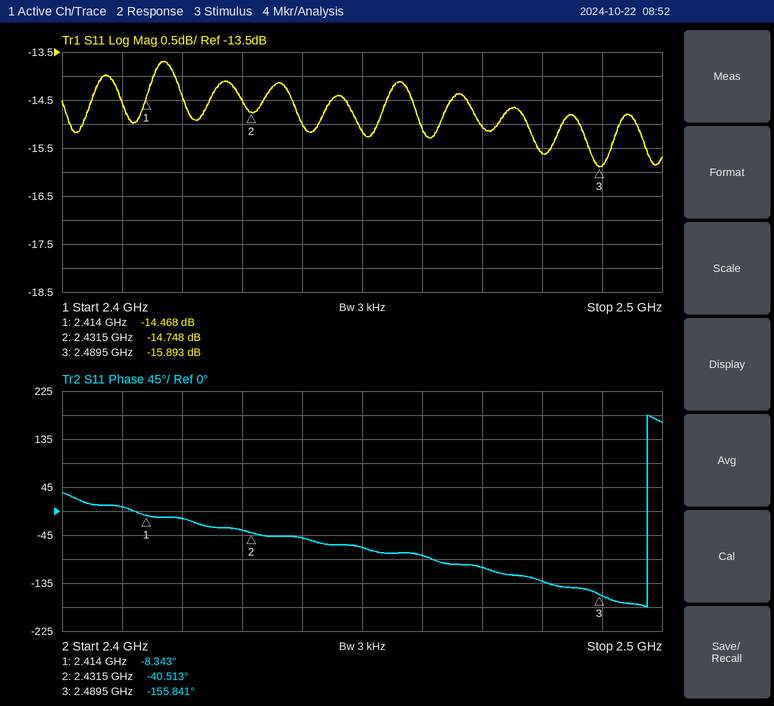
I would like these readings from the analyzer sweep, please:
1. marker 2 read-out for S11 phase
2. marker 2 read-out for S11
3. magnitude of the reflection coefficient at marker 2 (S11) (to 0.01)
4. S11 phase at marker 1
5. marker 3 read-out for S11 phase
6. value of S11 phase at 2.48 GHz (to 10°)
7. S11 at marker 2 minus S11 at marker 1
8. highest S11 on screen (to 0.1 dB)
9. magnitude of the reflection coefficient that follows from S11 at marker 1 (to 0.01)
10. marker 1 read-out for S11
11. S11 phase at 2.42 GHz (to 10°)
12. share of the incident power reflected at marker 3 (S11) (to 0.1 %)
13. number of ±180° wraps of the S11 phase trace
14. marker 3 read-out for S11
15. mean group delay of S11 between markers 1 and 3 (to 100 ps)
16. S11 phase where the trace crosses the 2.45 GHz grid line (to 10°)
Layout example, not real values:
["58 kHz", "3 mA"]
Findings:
["-40.513°", "-14.748 dB", "0.18", "-8.343°", "-155.841°", "-130°", "-0.280 dB", "-13.7 dB", "0.19", "-14.468 dB", "-10°", "2.6 %", "1", "-15.893 dB", "5.4 ns", "-70°"]
